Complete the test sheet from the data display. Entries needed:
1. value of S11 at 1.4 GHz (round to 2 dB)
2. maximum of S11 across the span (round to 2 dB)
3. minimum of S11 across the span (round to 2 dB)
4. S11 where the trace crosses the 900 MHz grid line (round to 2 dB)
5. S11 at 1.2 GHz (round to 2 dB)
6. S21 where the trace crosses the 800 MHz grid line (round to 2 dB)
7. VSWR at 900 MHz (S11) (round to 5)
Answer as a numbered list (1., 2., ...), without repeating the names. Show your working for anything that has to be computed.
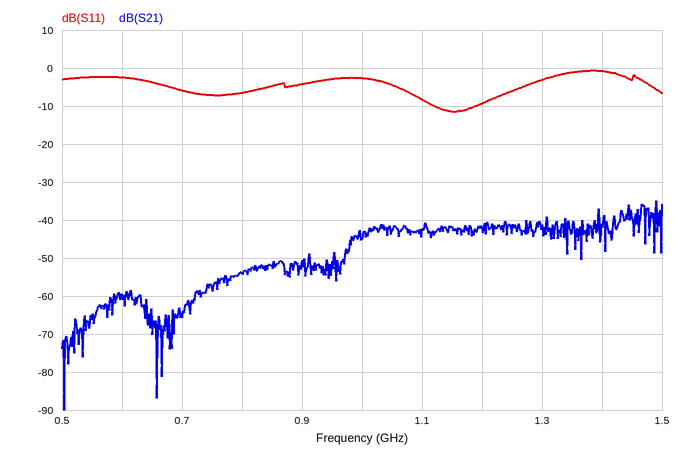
1. 0 dB
2. 0 dB
3. -12 dB
4. -4 dB
5. -10 dB
6. -54 dB
7. |Γ| = 10^(-4/20) = 0.6310; VSWR = (1 + 0.6310)/(1 − 0.6310) ≈ 4.42, so 5 to the nearest 5
